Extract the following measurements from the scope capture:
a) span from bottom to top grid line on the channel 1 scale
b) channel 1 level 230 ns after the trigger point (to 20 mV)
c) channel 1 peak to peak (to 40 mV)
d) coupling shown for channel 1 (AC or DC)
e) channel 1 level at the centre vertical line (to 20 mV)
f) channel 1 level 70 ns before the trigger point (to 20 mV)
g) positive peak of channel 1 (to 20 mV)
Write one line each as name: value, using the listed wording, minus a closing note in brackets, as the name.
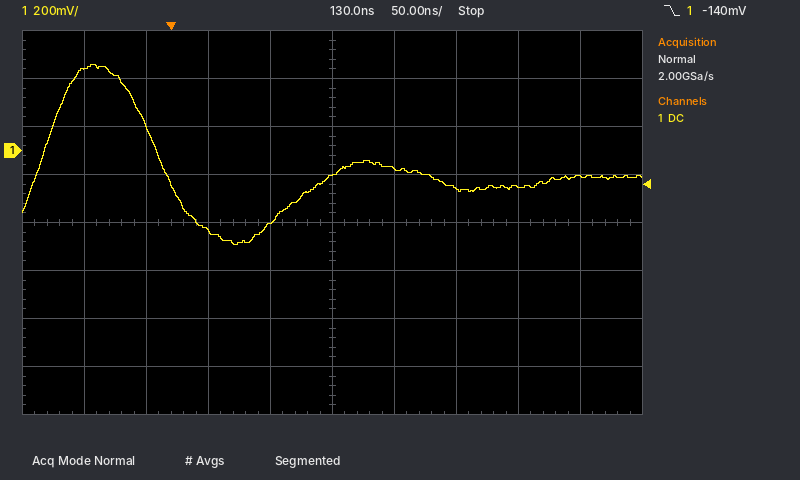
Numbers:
span from bottom to top grid line on the channel 1 scale: 1.6 V
channel 1 level 230 ns after the trigger point: -160 mV
channel 1 peak to peak: 760 mV
coupling shown for channel 1: DC
channel 1 level at the centre vertical line: -100 mV
channel 1 level 70 ns before the trigger point: 340 mV
positive peak of channel 1: 360 mV
